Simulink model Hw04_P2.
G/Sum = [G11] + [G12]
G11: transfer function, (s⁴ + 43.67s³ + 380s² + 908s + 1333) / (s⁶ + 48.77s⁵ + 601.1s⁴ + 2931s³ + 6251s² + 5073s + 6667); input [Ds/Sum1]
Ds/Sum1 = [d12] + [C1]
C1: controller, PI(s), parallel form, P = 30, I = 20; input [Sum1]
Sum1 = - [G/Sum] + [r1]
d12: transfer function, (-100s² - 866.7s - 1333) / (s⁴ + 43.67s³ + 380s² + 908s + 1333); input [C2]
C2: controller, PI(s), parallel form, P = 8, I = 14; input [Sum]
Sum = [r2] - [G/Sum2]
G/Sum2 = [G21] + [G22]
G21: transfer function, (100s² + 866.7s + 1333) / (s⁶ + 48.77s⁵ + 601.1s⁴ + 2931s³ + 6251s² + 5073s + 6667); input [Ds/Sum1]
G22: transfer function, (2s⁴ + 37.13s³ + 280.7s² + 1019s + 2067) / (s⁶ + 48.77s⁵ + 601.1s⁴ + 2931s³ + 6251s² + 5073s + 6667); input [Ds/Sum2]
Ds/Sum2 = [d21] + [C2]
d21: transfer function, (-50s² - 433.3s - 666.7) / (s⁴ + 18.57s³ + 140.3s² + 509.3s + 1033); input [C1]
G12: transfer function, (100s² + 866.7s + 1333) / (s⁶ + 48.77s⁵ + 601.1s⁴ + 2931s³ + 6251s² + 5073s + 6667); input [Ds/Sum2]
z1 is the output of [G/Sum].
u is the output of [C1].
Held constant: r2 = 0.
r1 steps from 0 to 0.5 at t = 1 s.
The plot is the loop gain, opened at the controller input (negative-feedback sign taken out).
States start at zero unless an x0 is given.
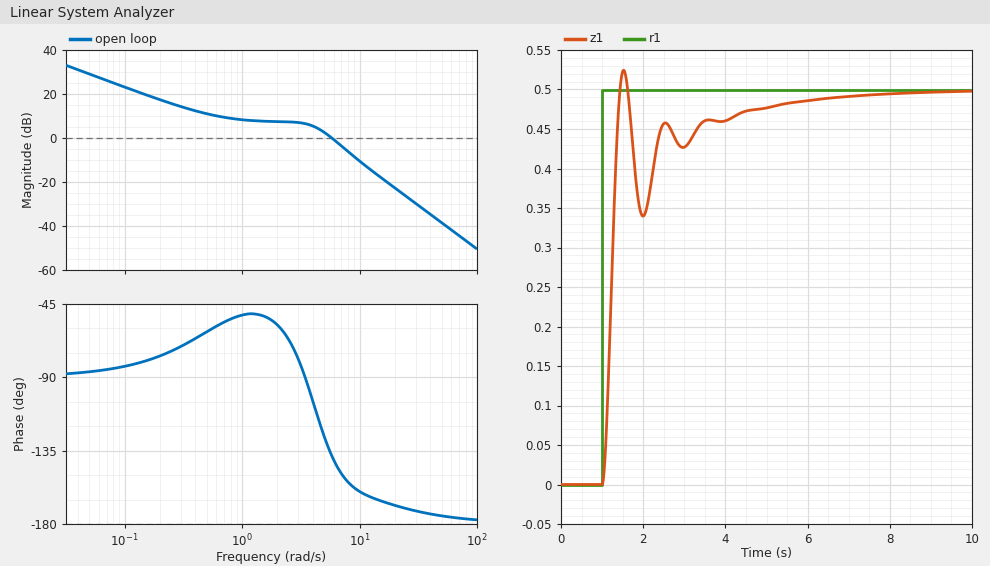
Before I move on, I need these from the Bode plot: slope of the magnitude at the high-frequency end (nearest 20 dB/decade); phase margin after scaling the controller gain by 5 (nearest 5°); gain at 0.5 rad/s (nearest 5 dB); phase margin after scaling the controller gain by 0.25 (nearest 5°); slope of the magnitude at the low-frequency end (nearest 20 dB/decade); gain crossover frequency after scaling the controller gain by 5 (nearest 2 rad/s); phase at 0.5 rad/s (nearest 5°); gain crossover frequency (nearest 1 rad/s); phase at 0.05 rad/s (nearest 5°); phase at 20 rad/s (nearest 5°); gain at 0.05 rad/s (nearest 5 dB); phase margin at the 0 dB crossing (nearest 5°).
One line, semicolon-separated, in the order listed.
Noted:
-40 dB/decade; 15°; 10 dB; 115°; -20 dB/decade; 12 rad/s; -60°; 6 rad/s; -85°; -170°; 30 dB; 40°
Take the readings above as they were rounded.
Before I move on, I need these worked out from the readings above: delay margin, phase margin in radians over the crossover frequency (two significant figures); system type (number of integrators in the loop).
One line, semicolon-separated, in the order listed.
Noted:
0.12 s; 1
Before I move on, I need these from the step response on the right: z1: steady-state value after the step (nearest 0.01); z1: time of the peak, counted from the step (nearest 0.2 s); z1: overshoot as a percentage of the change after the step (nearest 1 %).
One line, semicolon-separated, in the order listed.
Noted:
0.50; 0.6 s; 5 %
